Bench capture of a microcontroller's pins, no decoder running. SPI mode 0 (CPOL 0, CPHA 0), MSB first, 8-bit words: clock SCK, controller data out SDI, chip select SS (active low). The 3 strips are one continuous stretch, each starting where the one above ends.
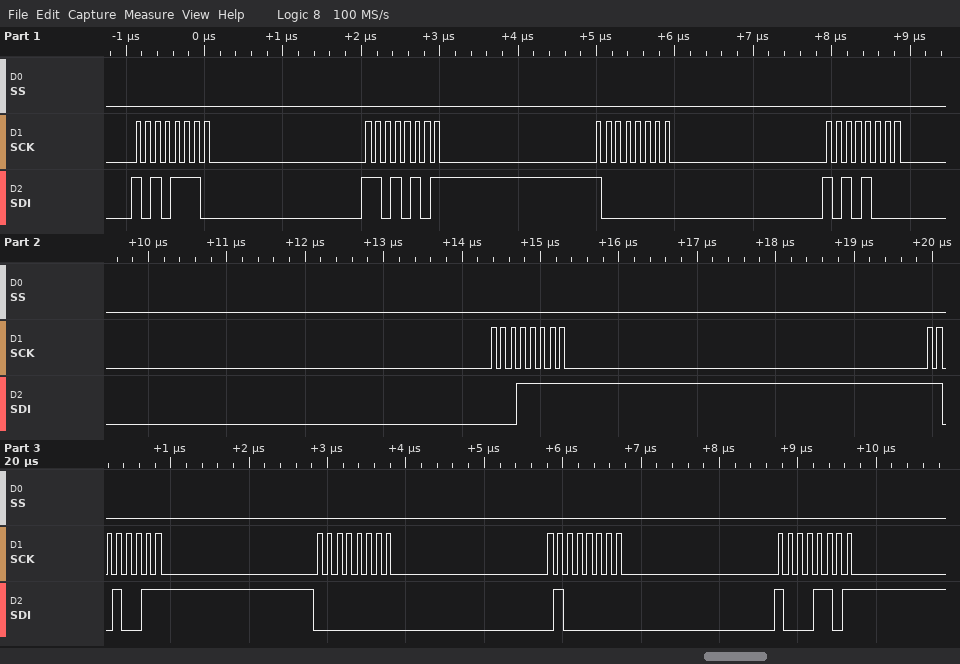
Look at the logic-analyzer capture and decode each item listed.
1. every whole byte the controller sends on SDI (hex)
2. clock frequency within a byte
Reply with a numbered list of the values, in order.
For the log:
1. 0xAE 0xD5 0x80 0xA8 0x1F 0xD3 0x00 0x40 0x8D
2. 8 MHz
